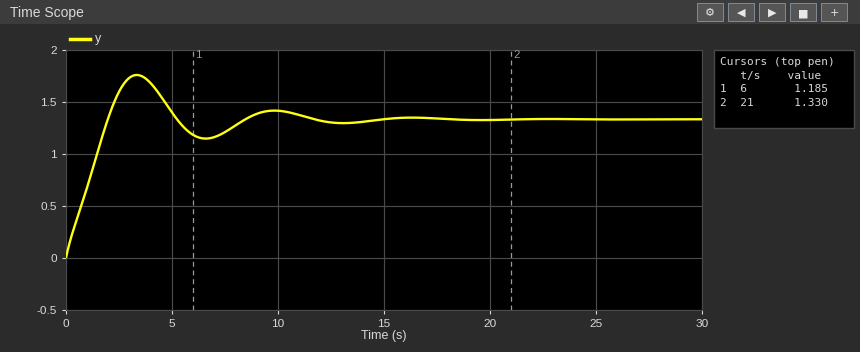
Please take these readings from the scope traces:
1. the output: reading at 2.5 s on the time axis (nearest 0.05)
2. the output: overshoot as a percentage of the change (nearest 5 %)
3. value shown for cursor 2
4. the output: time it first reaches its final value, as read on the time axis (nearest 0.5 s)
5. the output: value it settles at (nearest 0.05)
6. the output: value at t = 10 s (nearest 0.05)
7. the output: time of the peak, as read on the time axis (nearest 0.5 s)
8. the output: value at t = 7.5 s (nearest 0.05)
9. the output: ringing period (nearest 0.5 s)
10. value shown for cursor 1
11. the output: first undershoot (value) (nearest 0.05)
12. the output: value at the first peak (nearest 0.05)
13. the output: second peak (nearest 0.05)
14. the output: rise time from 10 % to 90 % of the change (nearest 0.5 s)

1.60
30 %
1.330
2.0 s
1.35
1.40
3.5 s
1.20
6.5 s
1.185
1.15
1.75
1.40
1.5 s
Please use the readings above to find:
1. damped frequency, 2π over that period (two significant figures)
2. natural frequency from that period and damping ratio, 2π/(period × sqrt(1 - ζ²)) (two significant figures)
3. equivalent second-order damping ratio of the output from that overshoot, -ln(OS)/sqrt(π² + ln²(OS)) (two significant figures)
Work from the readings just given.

0.97 rad/s
1.0 rad/s
0.36
